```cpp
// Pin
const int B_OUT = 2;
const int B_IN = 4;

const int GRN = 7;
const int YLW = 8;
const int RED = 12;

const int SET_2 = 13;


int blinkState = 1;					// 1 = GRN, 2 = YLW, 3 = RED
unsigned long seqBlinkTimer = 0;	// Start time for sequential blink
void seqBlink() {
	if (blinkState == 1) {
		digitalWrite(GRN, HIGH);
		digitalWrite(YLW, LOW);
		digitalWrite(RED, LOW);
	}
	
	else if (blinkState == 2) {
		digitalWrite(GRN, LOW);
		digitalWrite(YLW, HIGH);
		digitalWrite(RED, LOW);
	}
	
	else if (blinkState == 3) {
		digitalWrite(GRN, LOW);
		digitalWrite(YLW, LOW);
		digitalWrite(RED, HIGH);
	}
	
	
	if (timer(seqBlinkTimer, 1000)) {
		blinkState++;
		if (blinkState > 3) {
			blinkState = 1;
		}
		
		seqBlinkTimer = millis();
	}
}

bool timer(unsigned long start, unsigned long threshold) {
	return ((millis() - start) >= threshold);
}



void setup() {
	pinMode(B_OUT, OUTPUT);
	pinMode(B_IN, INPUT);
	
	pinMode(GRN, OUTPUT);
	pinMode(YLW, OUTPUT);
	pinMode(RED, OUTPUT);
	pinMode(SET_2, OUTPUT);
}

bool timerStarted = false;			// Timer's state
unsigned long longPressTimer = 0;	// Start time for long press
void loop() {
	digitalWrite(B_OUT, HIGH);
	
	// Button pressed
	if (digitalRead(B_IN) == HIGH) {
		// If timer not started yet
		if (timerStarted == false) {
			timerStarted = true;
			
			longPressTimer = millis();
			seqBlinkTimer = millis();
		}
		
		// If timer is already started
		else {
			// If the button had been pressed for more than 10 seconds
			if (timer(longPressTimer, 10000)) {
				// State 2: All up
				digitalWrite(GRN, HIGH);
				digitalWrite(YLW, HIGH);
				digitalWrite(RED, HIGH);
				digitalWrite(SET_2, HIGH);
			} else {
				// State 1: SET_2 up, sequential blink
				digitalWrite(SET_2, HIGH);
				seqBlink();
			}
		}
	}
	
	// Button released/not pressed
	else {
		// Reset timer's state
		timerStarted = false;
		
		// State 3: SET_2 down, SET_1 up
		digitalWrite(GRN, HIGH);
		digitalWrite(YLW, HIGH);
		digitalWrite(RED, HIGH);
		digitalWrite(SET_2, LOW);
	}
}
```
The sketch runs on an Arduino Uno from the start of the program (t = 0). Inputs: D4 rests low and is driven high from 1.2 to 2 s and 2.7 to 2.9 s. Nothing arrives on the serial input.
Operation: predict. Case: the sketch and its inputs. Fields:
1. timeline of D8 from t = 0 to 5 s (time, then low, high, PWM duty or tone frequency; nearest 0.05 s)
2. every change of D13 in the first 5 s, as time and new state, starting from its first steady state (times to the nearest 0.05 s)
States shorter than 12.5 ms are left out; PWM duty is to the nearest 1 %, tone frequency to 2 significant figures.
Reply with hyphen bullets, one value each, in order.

- 0 s high; 1.2 s low; 2 s high; 2.7 s low; 2.9 s high
- 0 s low; 1.2 s high; 2 s low; 2.7 s high; 2.9 s low
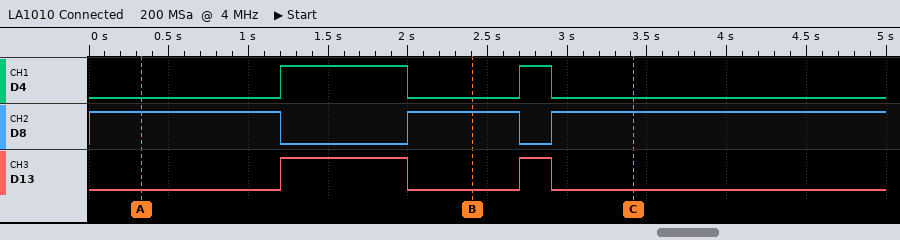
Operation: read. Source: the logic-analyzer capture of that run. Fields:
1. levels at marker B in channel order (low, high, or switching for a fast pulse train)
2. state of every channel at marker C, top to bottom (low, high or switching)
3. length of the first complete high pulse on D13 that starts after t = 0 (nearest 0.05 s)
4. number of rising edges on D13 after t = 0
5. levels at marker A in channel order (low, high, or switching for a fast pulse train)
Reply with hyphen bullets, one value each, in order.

- D4 low, D8 high, D13 low
- D4 low, D8 high, D13 low
- 0.80 s
- 2
- D4 low, D8 high, D13 low
